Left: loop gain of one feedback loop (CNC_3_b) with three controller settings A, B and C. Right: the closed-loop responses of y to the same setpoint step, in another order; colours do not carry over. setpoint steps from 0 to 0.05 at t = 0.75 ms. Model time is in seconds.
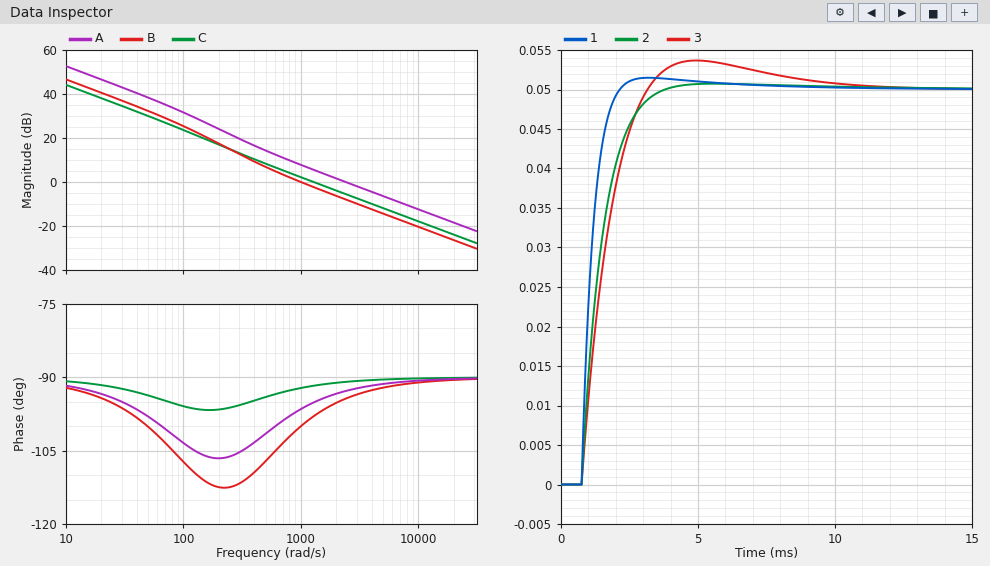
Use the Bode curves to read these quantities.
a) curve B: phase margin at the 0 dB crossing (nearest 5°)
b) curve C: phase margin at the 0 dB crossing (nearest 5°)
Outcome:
80°
90°
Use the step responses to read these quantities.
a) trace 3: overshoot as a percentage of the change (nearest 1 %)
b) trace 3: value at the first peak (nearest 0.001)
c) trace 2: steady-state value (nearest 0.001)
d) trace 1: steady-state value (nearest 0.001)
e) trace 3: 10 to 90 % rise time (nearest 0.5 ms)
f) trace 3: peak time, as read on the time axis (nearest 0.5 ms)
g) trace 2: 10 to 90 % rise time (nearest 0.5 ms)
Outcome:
7 %
0.054
0.050
0.050
1.5 ms
5.0 ms
1.5 ms
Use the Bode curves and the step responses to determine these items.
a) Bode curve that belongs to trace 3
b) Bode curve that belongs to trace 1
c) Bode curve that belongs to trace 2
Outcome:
B
A
C
